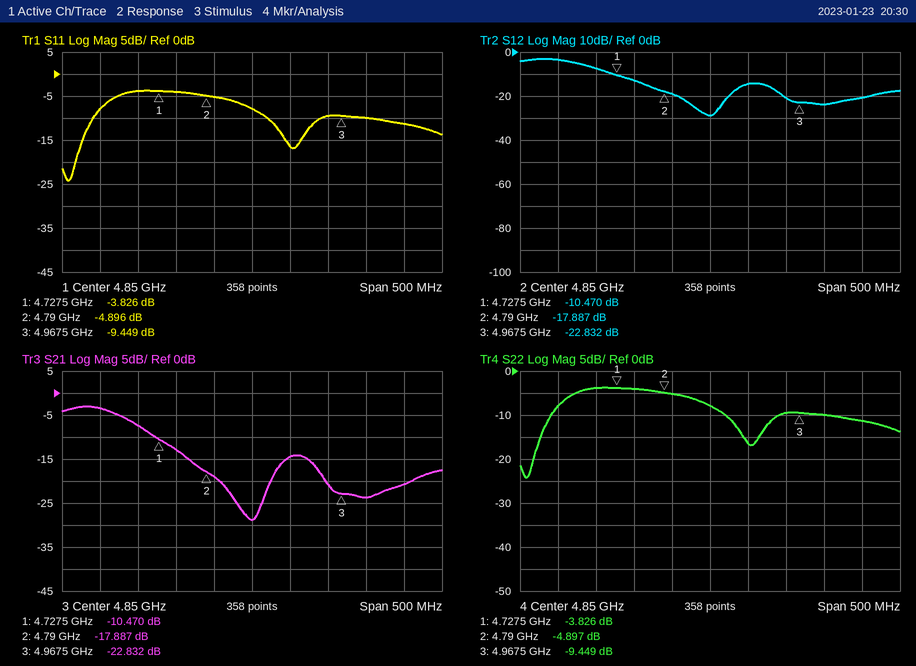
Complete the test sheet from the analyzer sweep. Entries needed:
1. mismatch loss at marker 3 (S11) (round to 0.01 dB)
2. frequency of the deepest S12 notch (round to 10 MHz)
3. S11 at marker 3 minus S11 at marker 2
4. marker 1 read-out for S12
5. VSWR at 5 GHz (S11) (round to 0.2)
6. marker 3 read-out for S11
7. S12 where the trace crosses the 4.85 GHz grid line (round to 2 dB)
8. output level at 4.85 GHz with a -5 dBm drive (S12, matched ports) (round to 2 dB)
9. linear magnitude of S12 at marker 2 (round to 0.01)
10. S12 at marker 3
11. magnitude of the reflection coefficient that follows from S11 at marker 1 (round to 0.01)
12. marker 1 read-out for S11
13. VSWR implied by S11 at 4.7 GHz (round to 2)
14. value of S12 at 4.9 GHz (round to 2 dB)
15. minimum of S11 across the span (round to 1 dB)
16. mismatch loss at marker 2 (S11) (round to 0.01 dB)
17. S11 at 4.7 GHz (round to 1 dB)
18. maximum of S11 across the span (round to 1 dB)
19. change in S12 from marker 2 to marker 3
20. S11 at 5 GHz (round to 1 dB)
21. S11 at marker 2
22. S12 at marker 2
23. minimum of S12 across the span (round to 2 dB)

0.52 dB
4.85 GHz
-4.553 dB
-10.470 dB
2.0
-9.449 dB
-28 dB
-34 dBm
0.13
-22.832 dB
0.64
-3.826 dB
4
-14 dB
-24 dB
1.70 dB
-4 dB
-4 dB
-4.945 dB
-10 dB
-4.896 dB
-17.887 dB
-28 dB
